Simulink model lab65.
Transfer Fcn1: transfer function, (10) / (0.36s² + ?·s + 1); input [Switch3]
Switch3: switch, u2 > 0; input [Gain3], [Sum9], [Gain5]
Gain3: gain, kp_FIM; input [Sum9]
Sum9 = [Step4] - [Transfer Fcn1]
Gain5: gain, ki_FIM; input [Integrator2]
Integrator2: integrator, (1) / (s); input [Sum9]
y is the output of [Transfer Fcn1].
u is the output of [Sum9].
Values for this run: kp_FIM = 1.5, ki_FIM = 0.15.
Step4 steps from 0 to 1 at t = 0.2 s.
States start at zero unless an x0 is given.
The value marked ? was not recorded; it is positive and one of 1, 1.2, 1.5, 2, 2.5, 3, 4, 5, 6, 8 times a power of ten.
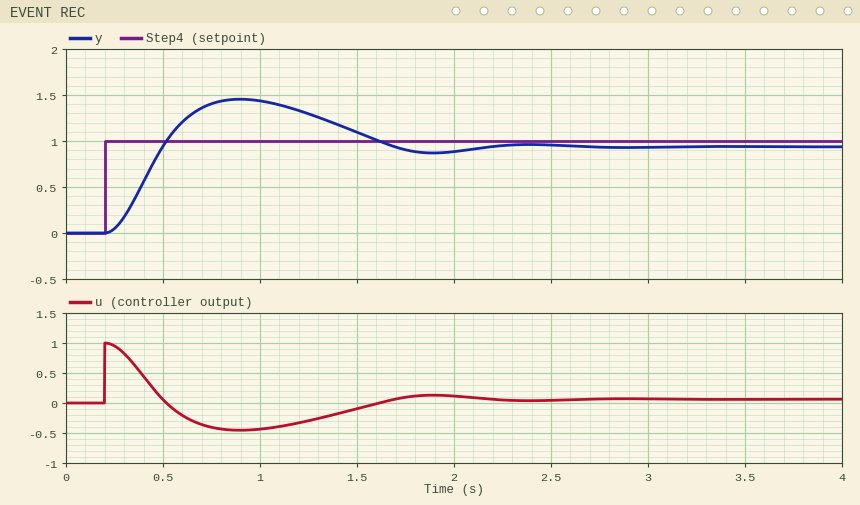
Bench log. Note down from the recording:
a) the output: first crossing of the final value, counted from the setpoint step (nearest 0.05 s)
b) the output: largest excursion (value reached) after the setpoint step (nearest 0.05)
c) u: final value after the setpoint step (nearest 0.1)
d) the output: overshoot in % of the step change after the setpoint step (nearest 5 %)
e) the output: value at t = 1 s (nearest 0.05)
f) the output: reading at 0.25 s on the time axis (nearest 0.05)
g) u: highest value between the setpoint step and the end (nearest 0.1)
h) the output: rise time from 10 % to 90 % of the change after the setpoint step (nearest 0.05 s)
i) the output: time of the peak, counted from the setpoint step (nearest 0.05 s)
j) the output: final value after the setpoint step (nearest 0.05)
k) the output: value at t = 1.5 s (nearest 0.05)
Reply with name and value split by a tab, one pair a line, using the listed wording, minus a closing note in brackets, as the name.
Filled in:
the output: first crossing of the final value, counted from the setpoint step	0.30 s
the output: largest excursion (value reached) after the setpoint step	1.45
u: final value after the setpoint step	0.1
the output: overshoot in % of the step change after the setpoint step	55 %
the output: value at t = 1 s	1.45
the output: reading at 0.25 s on the time axis	0.05
u: highest value between the setpoint step and the end	1.0
the output: rise time from 10 % to 90 % of the change after the setpoint step	0.20 s
the output: time of the peak, counted from the setpoint step	0.70 s
the output: final value after the setpoint step	0.95
the output: value at t = 1.5 s	1.10
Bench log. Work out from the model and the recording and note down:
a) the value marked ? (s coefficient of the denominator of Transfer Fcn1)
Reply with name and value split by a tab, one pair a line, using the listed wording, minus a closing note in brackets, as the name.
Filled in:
the value marked ?	1.5
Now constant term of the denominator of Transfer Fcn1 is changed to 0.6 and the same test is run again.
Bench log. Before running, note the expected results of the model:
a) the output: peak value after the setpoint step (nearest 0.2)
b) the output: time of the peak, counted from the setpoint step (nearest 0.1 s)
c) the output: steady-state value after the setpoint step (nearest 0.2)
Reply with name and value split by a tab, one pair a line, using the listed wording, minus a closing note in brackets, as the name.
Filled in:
the output: peak value after the setpoint step	1.6
the output: time of the peak, counted from the setpoint step	0.8 s
the output: steady-state value after the setpoint step	1.0
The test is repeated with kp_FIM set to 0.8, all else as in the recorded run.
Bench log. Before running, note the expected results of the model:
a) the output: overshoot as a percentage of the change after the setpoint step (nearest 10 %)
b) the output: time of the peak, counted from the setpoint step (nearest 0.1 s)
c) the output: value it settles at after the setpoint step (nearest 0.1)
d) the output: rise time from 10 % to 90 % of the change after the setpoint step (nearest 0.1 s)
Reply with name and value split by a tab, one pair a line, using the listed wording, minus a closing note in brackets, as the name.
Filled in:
the output: overshoot as a percentage of the change after the setpoint step	30 %
the output: time of the peak, counted from the setpoint step	0.8 s
the output: value it settles at after the setpoint step	0.9
the output: rise time from 10 % to 90 % of the change after the setpoint step	0.3 s
